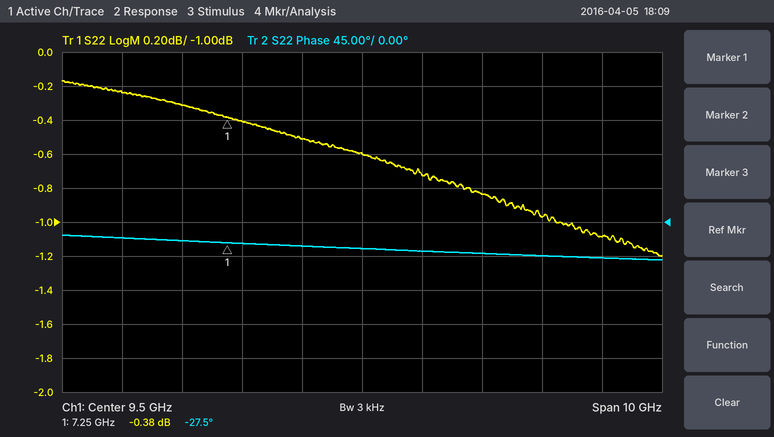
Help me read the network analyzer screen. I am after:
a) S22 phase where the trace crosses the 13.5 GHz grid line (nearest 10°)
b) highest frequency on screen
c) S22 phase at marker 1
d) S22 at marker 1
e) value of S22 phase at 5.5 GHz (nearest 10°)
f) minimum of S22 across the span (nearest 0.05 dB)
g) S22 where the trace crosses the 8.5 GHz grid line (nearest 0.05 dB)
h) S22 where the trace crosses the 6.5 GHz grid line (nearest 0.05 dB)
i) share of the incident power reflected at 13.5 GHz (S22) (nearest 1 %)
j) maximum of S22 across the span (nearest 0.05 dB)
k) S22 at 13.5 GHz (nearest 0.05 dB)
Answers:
-50°
14.5 GHz
-27.5°
-0.38 dB
-20°
-1.20 dB
-0.50 dB
-0.30 dB
78 %
-0.15 dB
-1.10 dB
